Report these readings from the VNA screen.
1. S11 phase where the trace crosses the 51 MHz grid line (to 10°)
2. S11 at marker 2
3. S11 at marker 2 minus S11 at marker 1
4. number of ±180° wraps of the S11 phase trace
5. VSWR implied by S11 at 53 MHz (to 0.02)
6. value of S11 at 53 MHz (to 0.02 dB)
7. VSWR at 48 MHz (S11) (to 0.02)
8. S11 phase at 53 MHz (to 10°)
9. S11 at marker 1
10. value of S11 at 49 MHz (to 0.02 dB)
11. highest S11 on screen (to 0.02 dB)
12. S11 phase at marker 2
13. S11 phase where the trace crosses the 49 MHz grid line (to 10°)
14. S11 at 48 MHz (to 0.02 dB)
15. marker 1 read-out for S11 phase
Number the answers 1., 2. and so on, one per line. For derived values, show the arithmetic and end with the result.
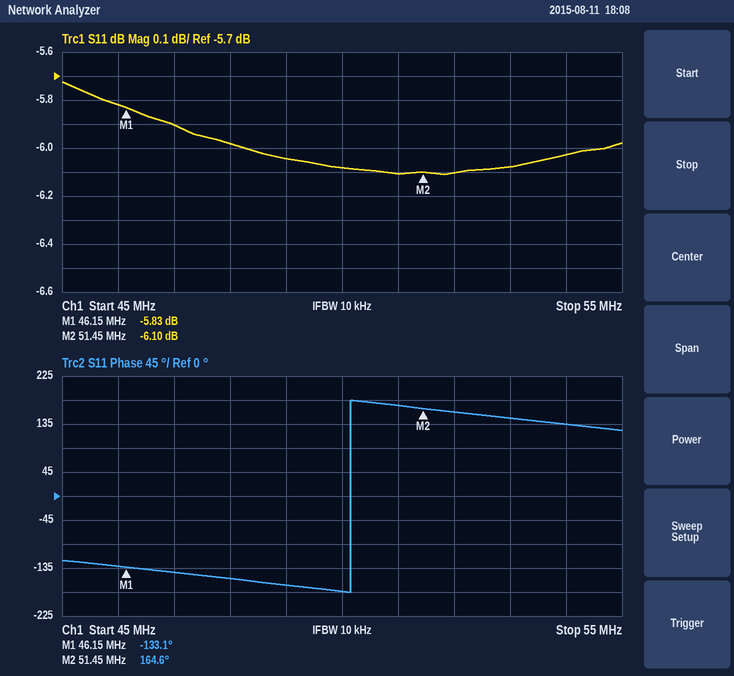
1. 170°
2. -6.10 dB
3. -6.1 − (-5.83) = -0.27 dB
4. 1
5. |Γ| = 10^(-6.08/20) = 0.4966; VSWR = (1 + 0.4966)/(1 − 0.4966) ≈ 2.97, so 2.98 to the nearest 0.02
6. -6.08 dB
7. |Γ| = 10^(-5.98/20) = 0.5023; VSWR = (1 + 0.5023)/(1 − 0.5023) ≈ 3.02
8. 150°
9. -5.83 dB
10. -6.04 dB
11. -5.72 dB
12. 164.6°
13. -170°
14. -5.98 dB
15. -133.1°
